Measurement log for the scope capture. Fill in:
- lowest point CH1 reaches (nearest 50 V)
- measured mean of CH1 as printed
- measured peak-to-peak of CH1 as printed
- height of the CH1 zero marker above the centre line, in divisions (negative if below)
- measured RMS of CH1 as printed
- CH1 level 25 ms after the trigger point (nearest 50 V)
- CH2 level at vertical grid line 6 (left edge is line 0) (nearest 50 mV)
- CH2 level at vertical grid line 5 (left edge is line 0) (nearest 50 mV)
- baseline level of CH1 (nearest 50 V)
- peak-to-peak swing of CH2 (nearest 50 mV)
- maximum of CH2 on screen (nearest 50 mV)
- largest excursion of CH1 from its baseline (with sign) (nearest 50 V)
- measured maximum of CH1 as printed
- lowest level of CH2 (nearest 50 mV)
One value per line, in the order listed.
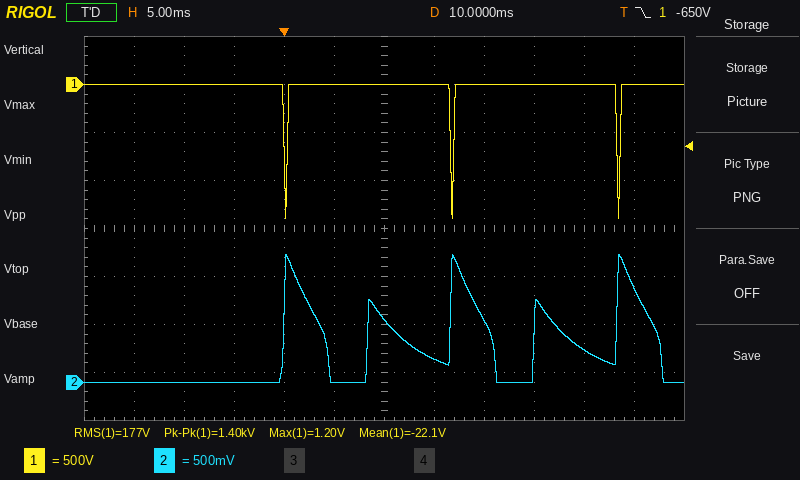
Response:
-1.40 kV
-22.1 V
1.40 kV
+3.0 div
177 V
0 V
650 mV
0 mV
0 V
1.35 V
1.35 V
-1.40 kV
1.20 V
0 mV
